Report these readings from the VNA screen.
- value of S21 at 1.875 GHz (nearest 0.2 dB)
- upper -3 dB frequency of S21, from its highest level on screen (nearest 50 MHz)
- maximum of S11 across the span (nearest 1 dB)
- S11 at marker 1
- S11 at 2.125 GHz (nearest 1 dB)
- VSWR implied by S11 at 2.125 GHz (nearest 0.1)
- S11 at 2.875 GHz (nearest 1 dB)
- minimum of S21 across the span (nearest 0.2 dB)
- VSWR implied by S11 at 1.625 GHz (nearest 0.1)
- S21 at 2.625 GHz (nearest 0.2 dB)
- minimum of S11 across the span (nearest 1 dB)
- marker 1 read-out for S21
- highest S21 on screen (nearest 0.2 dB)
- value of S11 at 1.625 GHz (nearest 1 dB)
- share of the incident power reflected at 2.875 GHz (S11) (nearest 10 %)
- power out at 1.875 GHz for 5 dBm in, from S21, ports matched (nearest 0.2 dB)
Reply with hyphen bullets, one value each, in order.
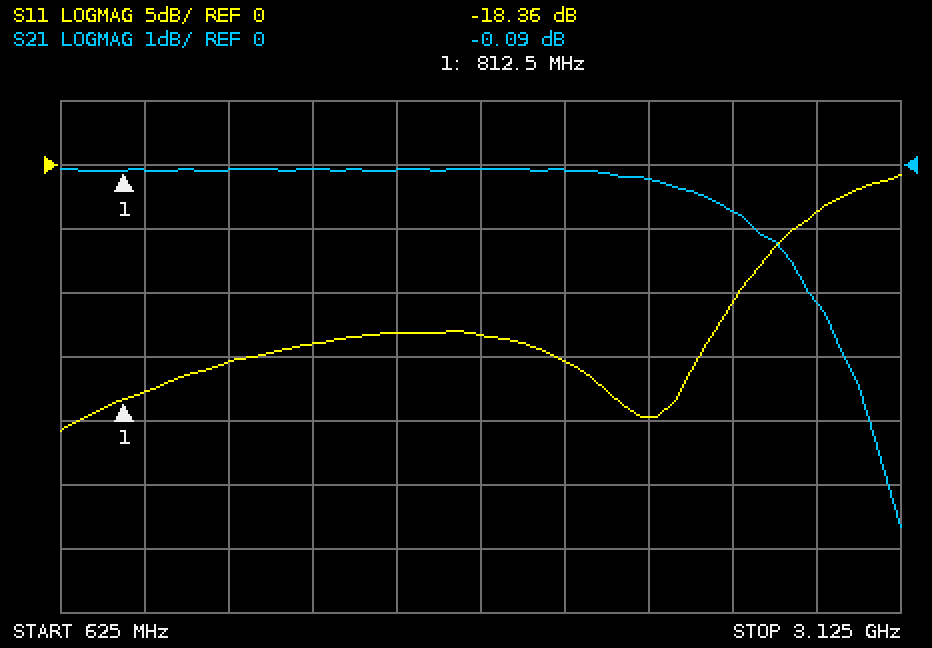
- 0.0 dB
- 2.95 GHz
- -1 dB
- -18.36 dB
- -15 dB
- 1.4
- -4 dB
- -5.6 dB
- 1.6
- -0.8 dB
- -21 dB
- -0.09 dB
- 0.0 dB
- -13 dB
- 40 %
- 5.0 dBm
